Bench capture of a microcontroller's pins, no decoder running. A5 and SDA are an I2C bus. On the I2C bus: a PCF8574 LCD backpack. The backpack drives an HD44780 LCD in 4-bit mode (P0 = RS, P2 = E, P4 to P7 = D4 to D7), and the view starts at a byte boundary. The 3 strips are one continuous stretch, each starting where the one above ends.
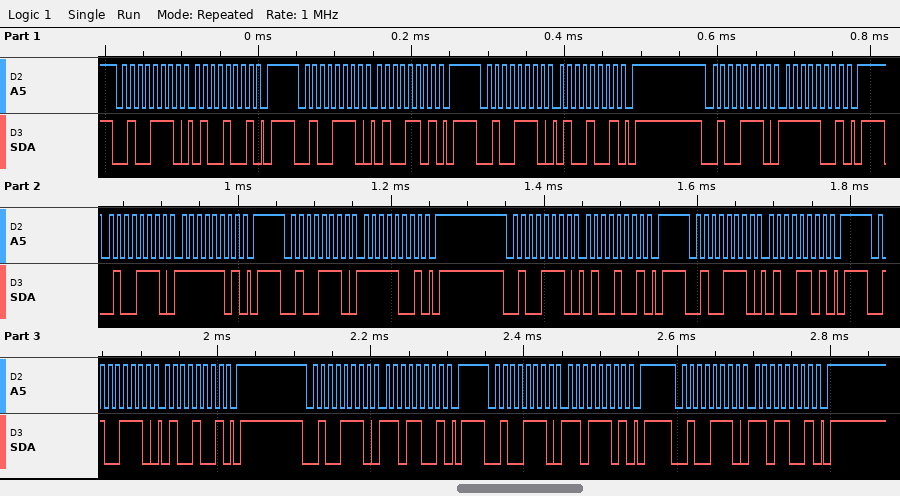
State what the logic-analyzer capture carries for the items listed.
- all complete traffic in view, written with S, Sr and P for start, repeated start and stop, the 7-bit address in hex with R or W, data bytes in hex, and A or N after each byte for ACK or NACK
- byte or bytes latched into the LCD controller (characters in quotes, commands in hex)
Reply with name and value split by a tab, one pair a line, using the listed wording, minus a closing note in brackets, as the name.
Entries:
all complete traffic in view, written with S, Sr and P for start, repeated start and stop, the 7-bit address in hex with R or W, data bytes in hex, and A or N after each byte for ACK or NACK	S 27W A 49 A P S 27W A 4D A P S 27W A 49 A P S 27W A F9 A P S 27W A FD A P S 27W A F9 A P S 27W A 49 A P S 27W A 4D A P S 27W A 49 A P S 27W A D9 A P S 27W A DD A P S 27W A D9 A P
byte or bytes latched into the LCD controller	'O' 'M'
